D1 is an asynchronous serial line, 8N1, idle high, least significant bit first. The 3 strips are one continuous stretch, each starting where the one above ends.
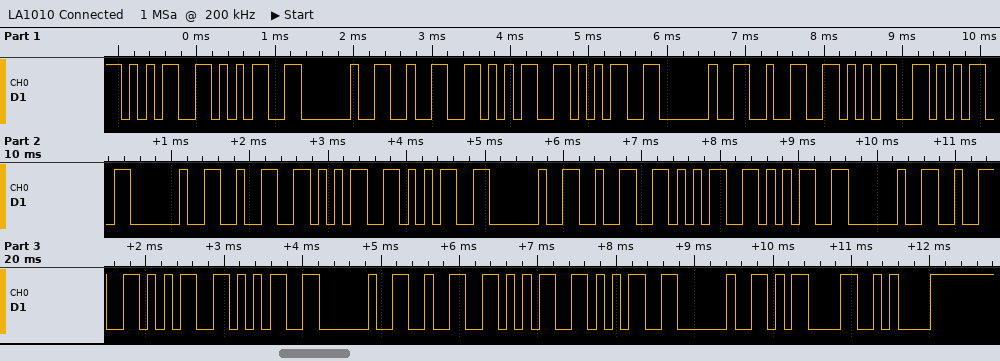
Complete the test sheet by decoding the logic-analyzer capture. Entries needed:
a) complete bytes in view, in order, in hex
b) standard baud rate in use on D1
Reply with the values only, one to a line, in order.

35 35 20 32 35 35 20 32 35 35 20 32 35 35 20 32 35 35 20 32 35 35 20 32 35 35 20 0D 0A
9600 baud
